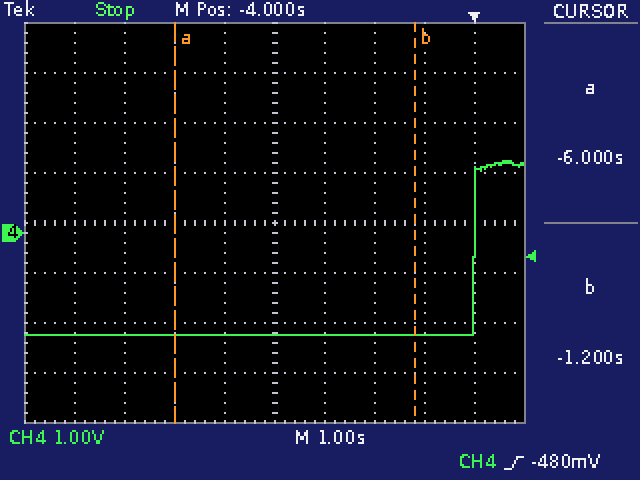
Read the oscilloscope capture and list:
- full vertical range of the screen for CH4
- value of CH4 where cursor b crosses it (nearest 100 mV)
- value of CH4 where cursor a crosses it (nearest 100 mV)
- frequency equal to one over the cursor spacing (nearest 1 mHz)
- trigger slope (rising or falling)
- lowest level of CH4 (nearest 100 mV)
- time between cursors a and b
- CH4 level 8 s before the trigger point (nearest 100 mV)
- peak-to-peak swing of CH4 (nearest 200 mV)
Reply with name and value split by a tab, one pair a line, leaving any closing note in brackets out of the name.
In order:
full vertical range of the screen for CH4	8 V
value of CH4 where cursor b crosses it	-2.0 V
value of CH4 where cursor a crosses it	-2.0 V
frequency equal to one over the cursor spacing	208 mHz
trigger slope	rising
lowest level of CH4	-2.0 V
time between cursors a and b	4.8 s
CH4 level 8 s before the trigger point	-2.0 V
peak-to-peak swing of CH4	3.4 V
